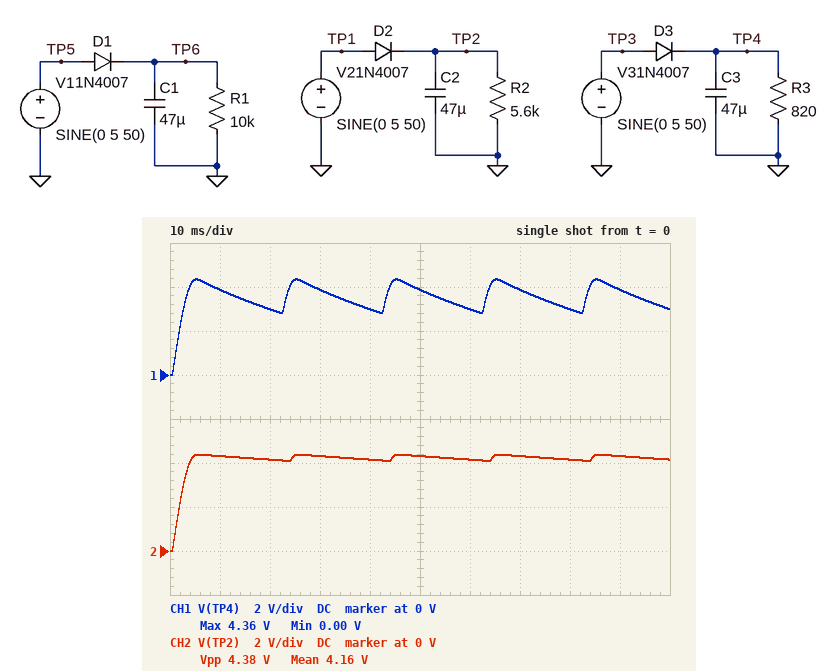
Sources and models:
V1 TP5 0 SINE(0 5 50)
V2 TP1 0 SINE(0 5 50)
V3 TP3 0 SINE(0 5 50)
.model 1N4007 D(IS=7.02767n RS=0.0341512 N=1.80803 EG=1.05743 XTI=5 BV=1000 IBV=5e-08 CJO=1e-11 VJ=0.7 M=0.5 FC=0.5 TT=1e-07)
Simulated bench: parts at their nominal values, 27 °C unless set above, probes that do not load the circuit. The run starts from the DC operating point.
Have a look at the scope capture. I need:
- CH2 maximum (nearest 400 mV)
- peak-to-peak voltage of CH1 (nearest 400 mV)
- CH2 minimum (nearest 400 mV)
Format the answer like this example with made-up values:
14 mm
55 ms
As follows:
4.4 V
4.4 V
0 V
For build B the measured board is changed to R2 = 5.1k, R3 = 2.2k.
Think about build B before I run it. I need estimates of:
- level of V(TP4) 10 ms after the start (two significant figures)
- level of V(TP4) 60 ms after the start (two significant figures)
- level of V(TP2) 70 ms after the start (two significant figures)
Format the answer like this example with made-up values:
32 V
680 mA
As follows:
4.2 V
3.8 V
4.3 V
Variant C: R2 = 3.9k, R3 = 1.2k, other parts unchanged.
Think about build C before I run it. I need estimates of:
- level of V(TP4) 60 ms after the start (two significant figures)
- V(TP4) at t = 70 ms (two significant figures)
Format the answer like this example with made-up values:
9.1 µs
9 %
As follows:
3.4 V
4.0 V
